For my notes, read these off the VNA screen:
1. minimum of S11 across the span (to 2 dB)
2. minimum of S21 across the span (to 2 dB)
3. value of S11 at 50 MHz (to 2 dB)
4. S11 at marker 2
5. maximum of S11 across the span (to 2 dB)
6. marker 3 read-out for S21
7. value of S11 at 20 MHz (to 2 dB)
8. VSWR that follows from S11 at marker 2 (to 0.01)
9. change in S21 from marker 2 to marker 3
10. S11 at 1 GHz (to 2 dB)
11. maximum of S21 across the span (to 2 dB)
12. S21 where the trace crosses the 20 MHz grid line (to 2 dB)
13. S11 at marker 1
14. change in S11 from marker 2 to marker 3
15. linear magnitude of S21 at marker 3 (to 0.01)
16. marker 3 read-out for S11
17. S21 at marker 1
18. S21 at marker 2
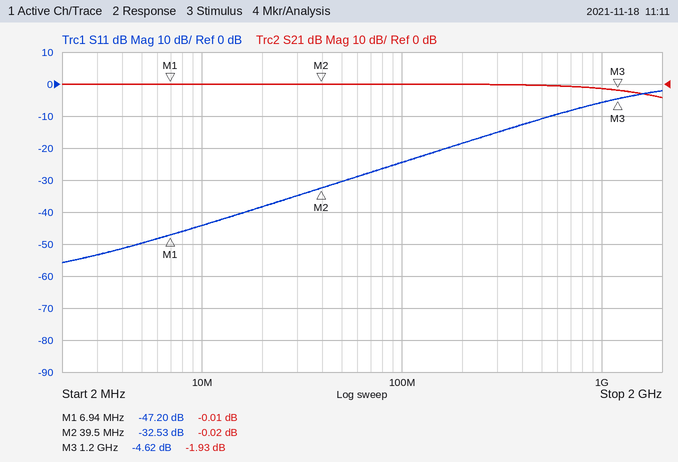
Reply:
-56 dB
-4 dB
-30 dB
-32.53 dB
-2 dB
-1.93 dB
-38 dB
1.05
-1.91 dB
-6 dB
0 dB
0 dB
-47.20 dB
27.91 dB
0.80
-4.62 dB
-0.01 dB
-0.02 dB
